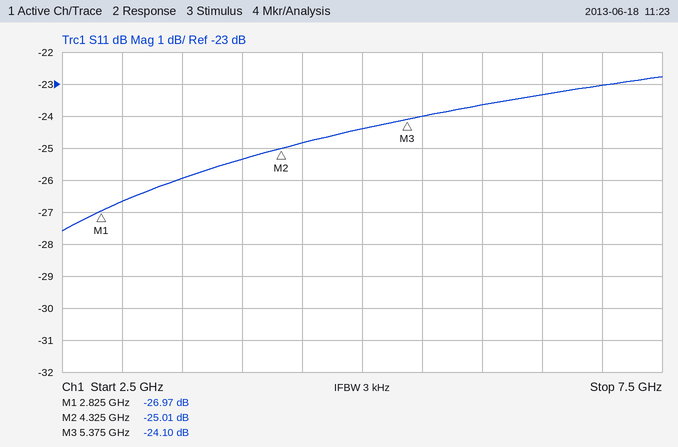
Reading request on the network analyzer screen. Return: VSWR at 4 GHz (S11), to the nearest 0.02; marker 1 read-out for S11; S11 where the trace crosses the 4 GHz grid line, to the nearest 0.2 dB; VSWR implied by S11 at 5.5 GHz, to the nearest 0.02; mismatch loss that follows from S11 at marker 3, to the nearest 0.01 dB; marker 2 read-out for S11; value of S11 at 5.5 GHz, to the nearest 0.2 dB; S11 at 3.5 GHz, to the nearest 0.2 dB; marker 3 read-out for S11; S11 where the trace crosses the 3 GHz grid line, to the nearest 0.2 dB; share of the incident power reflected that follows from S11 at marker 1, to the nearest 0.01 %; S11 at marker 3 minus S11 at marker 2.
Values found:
1.12
-26.97 dB
-25.4 dB
1.14
0.02 dB
-25.01 dB
-24.0 dB
-26.0 dB
-24.10 dB
-26.6 dB
0.20 %
0.91 dB
